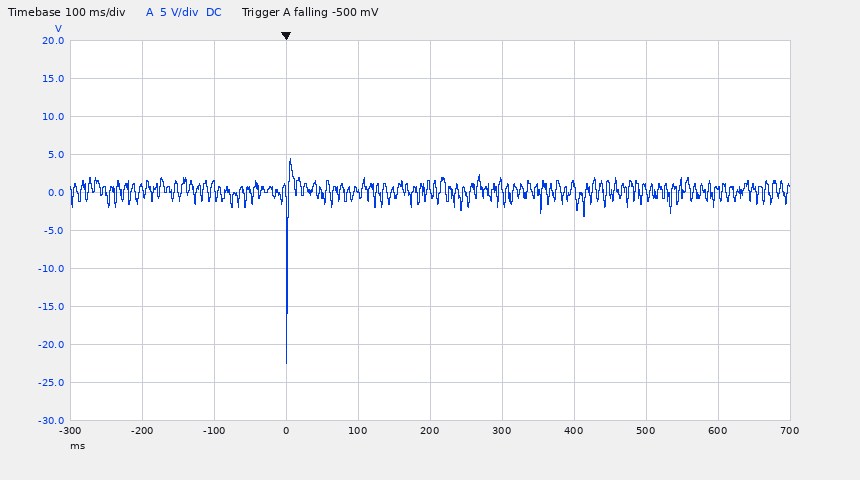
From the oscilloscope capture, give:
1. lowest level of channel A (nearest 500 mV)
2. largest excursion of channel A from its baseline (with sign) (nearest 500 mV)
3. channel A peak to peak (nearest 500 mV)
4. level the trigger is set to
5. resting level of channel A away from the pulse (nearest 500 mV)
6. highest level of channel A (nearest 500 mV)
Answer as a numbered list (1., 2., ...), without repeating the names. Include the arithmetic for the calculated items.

1. -22.5 V
2. -22.5 V − (500 mV) = -23.0 V
3. 4.5 V − (-22.5 V) = 27.0 V
4. -500 mV
5. 500 mV
6. 4.5 V
